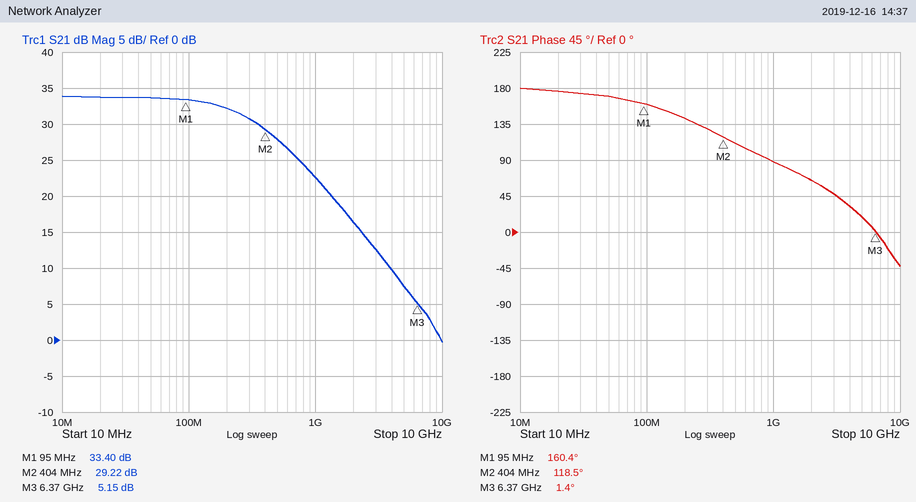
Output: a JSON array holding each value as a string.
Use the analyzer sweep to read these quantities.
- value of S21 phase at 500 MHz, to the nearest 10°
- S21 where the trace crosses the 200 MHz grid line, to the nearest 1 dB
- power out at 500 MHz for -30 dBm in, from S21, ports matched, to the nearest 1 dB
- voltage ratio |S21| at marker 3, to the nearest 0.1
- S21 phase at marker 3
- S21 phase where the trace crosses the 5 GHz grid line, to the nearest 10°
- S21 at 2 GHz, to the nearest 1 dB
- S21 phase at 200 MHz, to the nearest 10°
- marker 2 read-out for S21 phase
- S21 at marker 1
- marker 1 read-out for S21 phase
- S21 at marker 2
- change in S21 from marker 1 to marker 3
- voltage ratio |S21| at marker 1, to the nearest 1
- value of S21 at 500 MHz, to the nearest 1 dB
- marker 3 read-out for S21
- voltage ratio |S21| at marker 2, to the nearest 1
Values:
["110°", "32 dB", "-2 dBm", "1.8", "1.4°", "20°", "16 dB", "140°", "118.5°", "33.40 dB", "160.4°", "29.22 dB", "-28.25 dB", "47", "28 dB", "5.15 dB", "29"]
